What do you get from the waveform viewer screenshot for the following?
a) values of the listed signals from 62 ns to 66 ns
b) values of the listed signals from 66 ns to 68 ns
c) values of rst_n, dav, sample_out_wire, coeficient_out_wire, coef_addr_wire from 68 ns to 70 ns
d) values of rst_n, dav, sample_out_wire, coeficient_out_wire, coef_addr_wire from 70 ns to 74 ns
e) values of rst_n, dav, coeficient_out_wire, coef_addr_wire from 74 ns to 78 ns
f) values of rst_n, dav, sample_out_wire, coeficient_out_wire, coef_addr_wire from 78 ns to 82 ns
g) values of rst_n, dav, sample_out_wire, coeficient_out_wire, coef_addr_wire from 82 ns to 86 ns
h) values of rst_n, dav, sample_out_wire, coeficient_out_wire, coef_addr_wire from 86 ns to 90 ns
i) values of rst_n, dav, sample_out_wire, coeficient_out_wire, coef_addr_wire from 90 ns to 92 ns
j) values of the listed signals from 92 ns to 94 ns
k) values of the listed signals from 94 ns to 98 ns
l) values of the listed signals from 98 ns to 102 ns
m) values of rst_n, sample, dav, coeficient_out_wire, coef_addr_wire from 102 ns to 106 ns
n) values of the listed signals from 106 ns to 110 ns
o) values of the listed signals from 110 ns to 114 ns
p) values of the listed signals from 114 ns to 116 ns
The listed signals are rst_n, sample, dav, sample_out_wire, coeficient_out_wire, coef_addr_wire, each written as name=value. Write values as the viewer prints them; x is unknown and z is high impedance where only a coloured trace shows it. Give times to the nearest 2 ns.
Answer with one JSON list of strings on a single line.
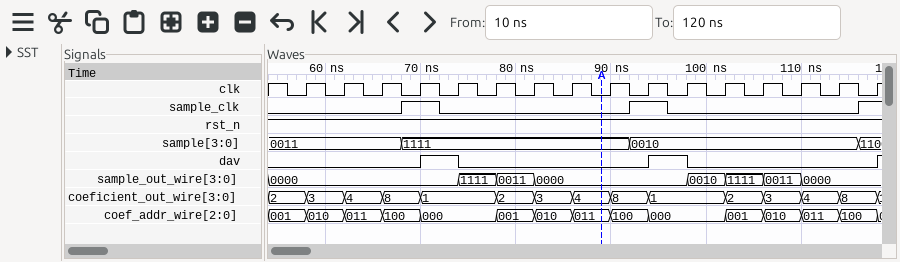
["rst_n=1, sample=0011, dav=0, sample_out_wire=0000, coeficient_out_wire=4, coef_addr_wire=011", "rst_n=1, sample=0011, dav=0, sample_out_wire=0000, coeficient_out_wire=8, coef_addr_wire=100", "rst_n=1, dav=0, sample_out_wire=0000, coeficient_out_wire=8, coef_addr_wire=100", "rst_n=1, dav=1, sample_out_wire=0000, coeficient_out_wire=1, coef_addr_wire=000", "rst_n=1, dav=0, coeficient_out_wire=1, coef_addr_wire=000", "rst_n=1, dav=0, sample_out_wire=0011, coeficient_out_wire=2, coef_addr_wire=001", "rst_n=1, dav=0, sample_out_wire=0000, coeficient_out_wire=3, coef_addr_wire=010", "rst_n=1, dav=0, sample_out_wire=0000, coeficient_out_wire=4, coef_addr_wire=011", "rst_n=1, dav=0, sample_out_wire=0000, coeficient_out_wire=8, coef_addr_wire=100", "rst_n=1, sample=0010, dav=0, sample_out_wire=0000, coeficient_out_wire=8, coef_addr_wire=100", "rst_n=1, sample=0010, dav=1, sample_out_wire=0000, coeficient_out_wire=1, coef_addr_wire=000", "rst_n=1, sample=0010, dav=0, sample_out_wire=0010, coeficient_out_wire=1, coef_addr_wire=000", "rst_n=1, sample=0010, dav=0, coeficient_out_wire=2, coef_addr_wire=001", "rst_n=1, sample=0010, dav=0, sample_out_wire=0011, coeficient_out_wire=3, coef_addr_wire=010", "rst_n=1, sample=0010, dav=0, sample_out_wire=0000, coeficient_out_wire=4, coef_addr_wire=011", "rst_n=1, sample=0010, dav=0, sample_out_wire=0000, coeficient_out_wire=8, coef_addr_wire=100"]
